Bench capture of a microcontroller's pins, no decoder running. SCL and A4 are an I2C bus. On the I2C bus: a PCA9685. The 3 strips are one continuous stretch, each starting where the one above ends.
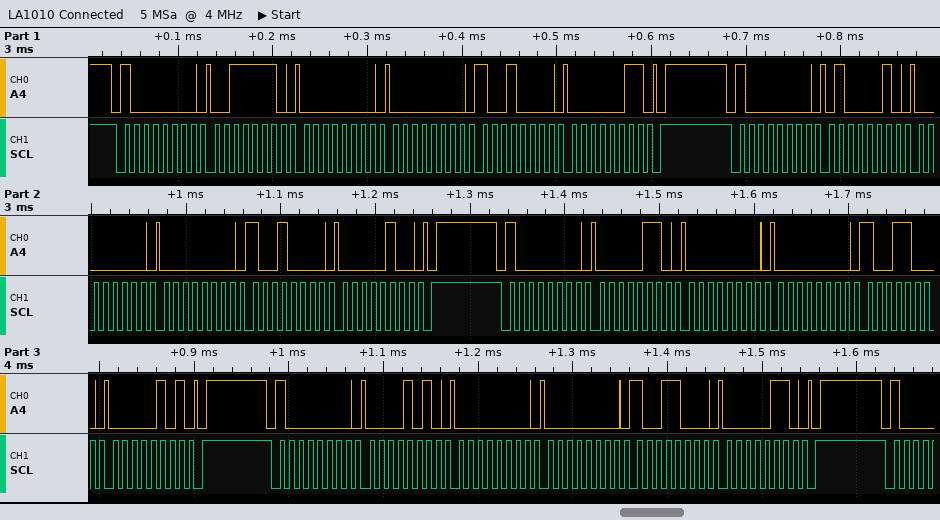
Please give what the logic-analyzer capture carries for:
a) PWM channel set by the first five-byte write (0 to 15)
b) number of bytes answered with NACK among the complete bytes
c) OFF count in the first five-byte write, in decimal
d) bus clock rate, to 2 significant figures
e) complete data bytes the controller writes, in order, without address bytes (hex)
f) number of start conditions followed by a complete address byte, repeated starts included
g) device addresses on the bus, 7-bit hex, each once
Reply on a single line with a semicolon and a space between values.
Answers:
14; 0; 912; 100 kHz; 3E 00 00 90 03 42 00 00 90 04 06 00 00 98 05 0A 00 00 98 06; 4; 0x40
